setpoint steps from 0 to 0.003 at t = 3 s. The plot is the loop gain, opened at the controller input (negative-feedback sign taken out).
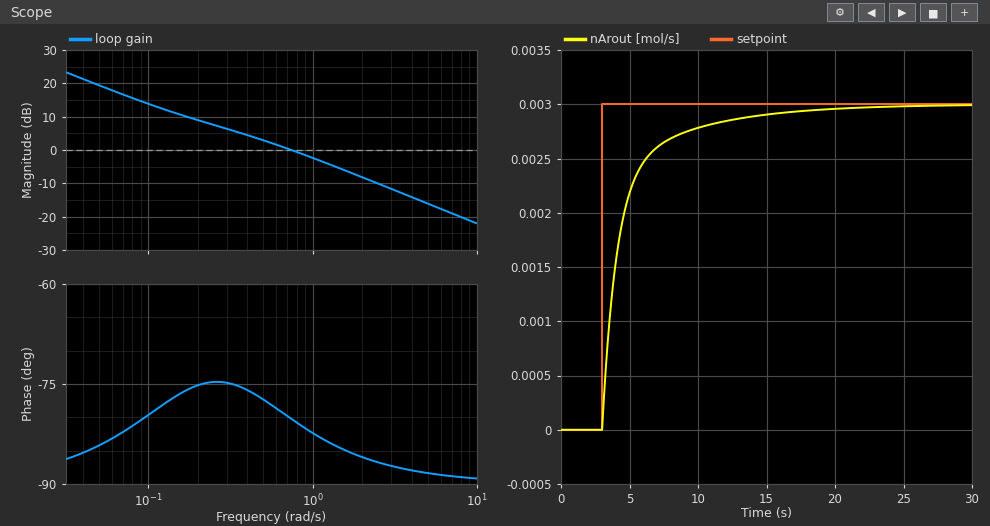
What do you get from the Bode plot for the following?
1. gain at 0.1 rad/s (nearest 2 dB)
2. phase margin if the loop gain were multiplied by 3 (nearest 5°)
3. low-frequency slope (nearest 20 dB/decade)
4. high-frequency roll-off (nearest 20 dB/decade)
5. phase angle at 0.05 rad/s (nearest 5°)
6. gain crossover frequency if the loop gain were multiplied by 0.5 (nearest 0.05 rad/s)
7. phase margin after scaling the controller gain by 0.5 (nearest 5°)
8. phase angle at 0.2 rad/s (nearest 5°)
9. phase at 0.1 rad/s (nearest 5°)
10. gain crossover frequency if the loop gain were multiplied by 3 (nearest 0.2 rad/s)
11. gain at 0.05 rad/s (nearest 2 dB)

14 dB
95°
-20 dB/decade
-20 dB/decade
-85°
0.30 rad/s
105°
-75°
-80°
2.4 rad/s
20 dB
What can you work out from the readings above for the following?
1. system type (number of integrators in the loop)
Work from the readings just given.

1
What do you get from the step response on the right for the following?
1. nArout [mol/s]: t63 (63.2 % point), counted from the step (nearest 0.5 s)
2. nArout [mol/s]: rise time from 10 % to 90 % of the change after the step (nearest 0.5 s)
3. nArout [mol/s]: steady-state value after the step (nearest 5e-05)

1.5 s
5.0 s
0.00300
